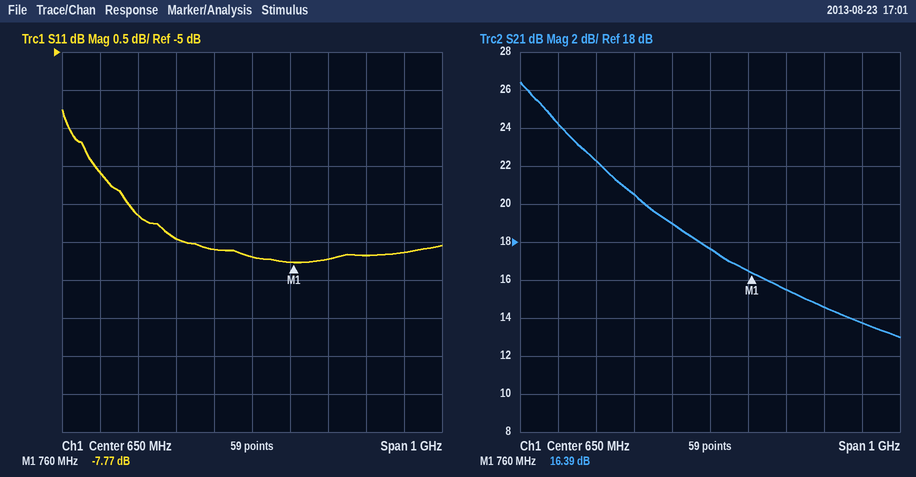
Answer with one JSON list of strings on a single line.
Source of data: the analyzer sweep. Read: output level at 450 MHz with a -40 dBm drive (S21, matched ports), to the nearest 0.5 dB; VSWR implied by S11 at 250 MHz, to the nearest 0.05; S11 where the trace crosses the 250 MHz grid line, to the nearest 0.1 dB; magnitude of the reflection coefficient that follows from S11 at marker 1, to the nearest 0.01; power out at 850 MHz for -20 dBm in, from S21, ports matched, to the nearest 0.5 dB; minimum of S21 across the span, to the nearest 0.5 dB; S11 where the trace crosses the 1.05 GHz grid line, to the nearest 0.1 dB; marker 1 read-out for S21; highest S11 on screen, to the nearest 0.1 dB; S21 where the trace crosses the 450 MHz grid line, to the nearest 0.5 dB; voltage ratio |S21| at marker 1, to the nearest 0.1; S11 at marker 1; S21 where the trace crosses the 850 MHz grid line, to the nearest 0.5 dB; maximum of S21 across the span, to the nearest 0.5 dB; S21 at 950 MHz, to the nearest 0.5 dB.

["-19.5 dBm", "2.75", "-6.6 dB", "0.41", "-4.5 dBm", "13.0 dB", "-7.6 dB", "16.39 dB", "-5.8 dB", "20.5 dB", "6.6", "-7.77 dB", "15.5 dB", "26.5 dB", "14.5 dB"]
